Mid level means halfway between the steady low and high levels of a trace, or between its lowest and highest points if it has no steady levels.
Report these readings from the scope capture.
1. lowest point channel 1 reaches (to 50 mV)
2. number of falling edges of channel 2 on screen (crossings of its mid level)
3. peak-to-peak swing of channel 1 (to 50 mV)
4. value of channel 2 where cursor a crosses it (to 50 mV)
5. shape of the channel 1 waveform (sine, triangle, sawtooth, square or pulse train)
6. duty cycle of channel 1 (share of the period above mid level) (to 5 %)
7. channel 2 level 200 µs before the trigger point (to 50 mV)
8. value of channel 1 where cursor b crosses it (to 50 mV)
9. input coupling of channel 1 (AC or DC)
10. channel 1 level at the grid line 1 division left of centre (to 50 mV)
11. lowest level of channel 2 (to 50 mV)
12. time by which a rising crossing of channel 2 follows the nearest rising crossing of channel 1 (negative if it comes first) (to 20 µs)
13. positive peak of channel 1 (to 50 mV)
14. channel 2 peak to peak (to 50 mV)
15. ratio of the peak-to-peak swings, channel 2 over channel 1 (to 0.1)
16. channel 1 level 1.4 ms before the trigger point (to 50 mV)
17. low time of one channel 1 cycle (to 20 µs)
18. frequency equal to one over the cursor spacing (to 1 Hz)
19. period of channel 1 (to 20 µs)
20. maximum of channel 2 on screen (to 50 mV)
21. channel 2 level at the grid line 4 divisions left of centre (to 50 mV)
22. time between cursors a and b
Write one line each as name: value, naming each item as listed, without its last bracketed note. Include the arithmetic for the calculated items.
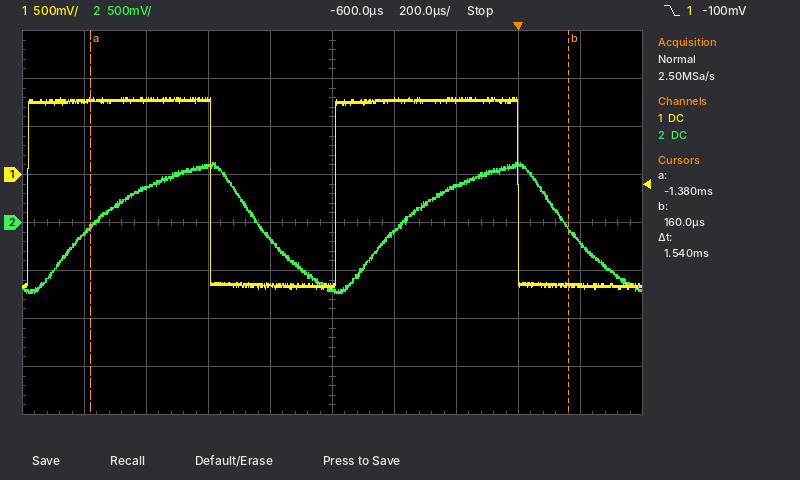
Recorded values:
lowest point channel 1 reaches: -1.20 V
number of falling edges of channel 2 on screen: 2
peak-to-peak swing of channel 1: 800 mV − (-1.20 V) = 2.00 V
value of channel 2 where cursor a crosses it: -50 mV
shape of the channel 1 waveform: pulse train
duty cycle of channel 1 (share of the period above mid level): 60 %
channel 2 level 200 µs before the trigger point: 350 mV
value of channel 1 where cursor b crosses it: -1.15 V
input coupling of channel 1: DC
channel 1 level at the grid line 1 division left of centre: -1.15 V
lowest level of channel 2: -750 mV
time by which a rising crossing of channel 2 follows the nearest rising crossing of channel 1 (negative if it comes first): +200 µs
positive peak of channel 1: 800 mV
channel 2 peak to peak: 600 mV − (-750 mV) = 1.35 V
ratio of the peak-to-peak swings, channel 2 over channel 1: 1.35 V / 2.00 V ≈ 0.7
channel 1 level 1.4 ms before the trigger point: 750 mV
low time of one channel 1 cycle: 400 µs
frequency equal to one over the cursor spacing: 1 / 1.54 ms ≈ 649 Hz
period of channel 1: 1.00 ms
maximum of channel 2 on screen: 600 mV
channel 2 level at the grid line 4 divisions left of centre: -100 mV
time between cursors a and b: 1.54 ms
